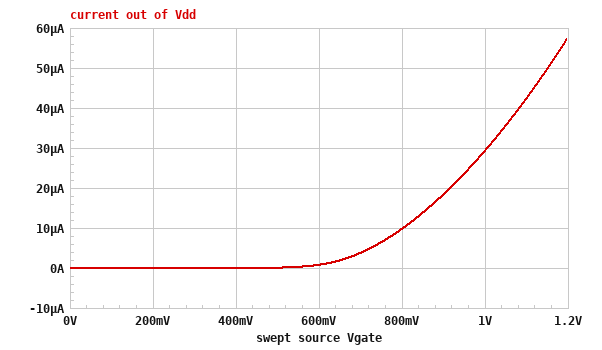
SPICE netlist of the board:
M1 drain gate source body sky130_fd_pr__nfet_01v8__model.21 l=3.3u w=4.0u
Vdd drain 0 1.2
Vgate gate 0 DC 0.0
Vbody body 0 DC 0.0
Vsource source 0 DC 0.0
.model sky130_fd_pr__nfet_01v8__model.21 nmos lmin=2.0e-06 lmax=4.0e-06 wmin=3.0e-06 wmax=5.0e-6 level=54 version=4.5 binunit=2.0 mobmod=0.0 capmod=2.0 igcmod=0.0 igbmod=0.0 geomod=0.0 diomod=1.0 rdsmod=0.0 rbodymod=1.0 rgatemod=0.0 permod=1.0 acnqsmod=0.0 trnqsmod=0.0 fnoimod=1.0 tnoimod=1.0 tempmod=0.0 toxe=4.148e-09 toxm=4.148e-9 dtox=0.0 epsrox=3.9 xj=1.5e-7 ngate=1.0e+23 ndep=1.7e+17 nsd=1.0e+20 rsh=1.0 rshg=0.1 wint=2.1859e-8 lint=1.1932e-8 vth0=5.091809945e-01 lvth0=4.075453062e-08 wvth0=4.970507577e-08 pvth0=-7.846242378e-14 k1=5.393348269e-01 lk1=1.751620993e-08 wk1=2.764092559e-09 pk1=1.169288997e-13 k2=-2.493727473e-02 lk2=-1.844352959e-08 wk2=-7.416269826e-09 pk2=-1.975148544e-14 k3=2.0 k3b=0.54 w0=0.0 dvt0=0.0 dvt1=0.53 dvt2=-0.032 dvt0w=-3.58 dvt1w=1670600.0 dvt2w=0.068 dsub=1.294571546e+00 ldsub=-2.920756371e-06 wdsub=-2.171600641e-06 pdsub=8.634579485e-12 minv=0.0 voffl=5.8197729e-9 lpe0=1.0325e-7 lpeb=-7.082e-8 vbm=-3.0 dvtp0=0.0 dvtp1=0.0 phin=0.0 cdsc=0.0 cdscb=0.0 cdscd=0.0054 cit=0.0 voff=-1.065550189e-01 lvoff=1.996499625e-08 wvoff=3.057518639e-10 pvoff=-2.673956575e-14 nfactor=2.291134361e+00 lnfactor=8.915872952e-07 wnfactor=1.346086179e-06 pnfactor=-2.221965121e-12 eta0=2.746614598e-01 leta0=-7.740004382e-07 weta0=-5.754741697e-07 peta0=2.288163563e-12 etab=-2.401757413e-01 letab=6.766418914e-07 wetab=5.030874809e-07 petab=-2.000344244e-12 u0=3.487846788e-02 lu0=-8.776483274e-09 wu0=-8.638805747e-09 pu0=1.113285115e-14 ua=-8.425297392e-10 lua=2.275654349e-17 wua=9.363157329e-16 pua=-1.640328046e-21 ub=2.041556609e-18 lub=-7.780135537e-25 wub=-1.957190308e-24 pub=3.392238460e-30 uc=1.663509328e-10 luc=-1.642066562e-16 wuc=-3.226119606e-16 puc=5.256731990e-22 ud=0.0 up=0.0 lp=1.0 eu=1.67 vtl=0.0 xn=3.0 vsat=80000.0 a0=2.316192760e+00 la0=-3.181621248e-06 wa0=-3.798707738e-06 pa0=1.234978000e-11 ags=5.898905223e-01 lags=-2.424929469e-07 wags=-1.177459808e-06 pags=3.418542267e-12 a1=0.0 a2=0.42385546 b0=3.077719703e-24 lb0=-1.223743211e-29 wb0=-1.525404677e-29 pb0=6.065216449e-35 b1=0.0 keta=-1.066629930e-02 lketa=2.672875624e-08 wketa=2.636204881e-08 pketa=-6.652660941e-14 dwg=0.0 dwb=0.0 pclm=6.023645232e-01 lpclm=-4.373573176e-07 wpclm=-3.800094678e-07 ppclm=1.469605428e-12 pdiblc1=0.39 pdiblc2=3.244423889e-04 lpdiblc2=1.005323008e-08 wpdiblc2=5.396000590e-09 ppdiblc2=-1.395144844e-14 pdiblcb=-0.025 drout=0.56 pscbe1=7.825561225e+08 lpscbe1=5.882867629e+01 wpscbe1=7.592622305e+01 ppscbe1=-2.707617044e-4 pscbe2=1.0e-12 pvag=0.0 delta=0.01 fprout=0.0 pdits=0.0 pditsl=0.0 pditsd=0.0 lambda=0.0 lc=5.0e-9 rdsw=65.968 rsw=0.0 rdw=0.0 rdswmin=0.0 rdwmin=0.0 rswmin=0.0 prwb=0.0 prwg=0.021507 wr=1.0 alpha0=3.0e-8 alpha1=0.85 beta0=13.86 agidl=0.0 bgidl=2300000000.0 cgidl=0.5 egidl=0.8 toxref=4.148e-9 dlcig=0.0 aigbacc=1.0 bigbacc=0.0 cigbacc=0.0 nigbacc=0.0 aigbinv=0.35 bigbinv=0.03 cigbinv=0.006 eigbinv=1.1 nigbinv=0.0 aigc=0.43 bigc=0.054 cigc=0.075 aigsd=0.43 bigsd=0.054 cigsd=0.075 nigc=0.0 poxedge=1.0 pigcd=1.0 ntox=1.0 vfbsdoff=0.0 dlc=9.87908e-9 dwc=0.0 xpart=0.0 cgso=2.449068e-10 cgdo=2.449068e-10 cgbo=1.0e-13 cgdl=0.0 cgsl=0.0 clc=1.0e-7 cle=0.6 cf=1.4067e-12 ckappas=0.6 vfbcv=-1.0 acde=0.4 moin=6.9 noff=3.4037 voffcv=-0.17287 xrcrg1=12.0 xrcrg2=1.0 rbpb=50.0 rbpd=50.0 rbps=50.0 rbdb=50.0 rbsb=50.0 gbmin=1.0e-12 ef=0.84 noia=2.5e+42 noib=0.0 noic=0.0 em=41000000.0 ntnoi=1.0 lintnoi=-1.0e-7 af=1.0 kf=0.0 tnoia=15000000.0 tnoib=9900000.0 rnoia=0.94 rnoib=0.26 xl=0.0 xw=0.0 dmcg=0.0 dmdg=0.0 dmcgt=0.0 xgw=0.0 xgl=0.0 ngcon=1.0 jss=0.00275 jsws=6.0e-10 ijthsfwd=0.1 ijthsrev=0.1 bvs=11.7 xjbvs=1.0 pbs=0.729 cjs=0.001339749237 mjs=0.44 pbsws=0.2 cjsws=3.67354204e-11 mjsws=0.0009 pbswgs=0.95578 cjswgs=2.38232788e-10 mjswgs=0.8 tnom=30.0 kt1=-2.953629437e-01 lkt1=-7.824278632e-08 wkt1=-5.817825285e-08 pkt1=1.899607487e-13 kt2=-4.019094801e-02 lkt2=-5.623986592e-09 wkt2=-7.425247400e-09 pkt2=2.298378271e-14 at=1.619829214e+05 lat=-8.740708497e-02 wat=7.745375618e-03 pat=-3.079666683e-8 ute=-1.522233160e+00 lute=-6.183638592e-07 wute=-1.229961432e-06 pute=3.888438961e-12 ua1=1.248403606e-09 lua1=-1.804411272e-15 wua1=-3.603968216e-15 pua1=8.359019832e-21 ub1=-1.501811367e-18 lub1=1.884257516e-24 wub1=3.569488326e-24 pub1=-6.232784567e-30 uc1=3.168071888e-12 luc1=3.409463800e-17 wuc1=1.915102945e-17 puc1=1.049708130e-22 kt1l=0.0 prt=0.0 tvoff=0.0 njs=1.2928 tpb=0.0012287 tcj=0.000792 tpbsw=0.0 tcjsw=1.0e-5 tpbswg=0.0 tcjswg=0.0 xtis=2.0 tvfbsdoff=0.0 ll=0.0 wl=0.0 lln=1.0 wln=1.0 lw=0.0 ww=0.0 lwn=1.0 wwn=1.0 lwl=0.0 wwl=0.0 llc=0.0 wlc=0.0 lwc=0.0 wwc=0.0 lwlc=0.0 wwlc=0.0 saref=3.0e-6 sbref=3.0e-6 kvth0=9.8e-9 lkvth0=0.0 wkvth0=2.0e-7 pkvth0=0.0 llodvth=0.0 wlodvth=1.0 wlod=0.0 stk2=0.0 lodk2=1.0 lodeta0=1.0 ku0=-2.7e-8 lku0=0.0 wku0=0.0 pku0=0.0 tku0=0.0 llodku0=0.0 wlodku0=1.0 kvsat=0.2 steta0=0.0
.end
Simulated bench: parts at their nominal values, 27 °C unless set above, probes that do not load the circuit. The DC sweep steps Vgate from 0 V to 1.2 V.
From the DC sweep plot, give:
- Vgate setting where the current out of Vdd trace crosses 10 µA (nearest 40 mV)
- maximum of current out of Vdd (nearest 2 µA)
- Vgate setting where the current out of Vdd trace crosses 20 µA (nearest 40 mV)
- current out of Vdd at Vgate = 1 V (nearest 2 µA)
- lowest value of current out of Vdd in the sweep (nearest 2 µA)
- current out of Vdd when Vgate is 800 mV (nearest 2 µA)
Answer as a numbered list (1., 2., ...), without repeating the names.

1. 800 mV
2. 58 µA
3. 920 mV
4. 30 µA
5. 0 A
6. 10 µA
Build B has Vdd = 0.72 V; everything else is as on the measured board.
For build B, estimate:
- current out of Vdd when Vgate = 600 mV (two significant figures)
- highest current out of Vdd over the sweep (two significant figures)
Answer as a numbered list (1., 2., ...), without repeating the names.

1. 790 nA
2. 57 µA
